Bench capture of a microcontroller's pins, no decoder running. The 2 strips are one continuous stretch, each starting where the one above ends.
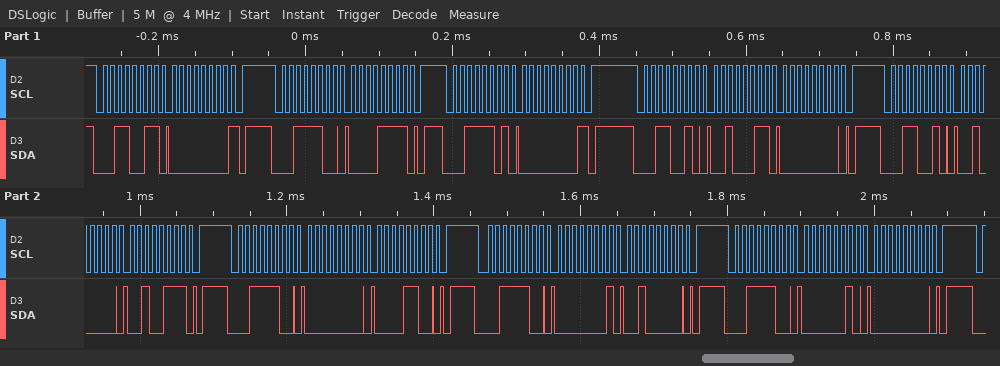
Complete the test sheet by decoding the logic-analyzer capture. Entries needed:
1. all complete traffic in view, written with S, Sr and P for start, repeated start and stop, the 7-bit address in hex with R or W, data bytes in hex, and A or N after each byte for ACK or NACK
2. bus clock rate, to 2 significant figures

S 19R A 00 N P S 1EW A 0F A P S 1ER A 00 N P S 19W A 23 A 00 A P S 19W A 20 A 27 A P S 1EW A 00 A 0C A P S 1EW A 01 A 20 A P S 1EW A 02 A 00 A P
100 kHz
